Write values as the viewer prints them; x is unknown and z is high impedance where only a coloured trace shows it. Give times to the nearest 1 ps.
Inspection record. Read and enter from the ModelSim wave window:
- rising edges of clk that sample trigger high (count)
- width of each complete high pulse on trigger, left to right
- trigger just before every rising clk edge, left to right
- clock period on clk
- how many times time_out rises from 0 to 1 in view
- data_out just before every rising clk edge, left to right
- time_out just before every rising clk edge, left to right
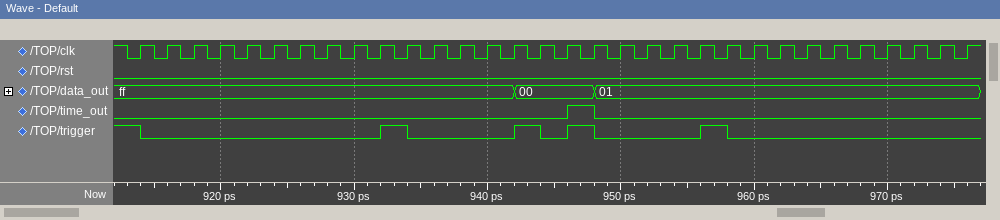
5
2 ps, 2 ps, 2 ps, 2 ps
1 0 0 0 0 0 0 0 0 0 1 0 0 0 0 1 0 1 0 0 0 0 1 0 0 0 0 0 0 0 0 0
2 ps
1
ff, ff, ff, ff, ff, ff, ff, ff, ff, ff, ff, ff, ff, ff, ff, 00, 00, 00, 01, 01, 01, 01, 01, 01, 01, 01, 01, 01, 01, 01, 01, 01
0 0 0 0 0 0 0 0 0 0 0 0 0 0 0 0 0 1 0 0 0 0 0 0 0 0 0 0 0 0 0 0
